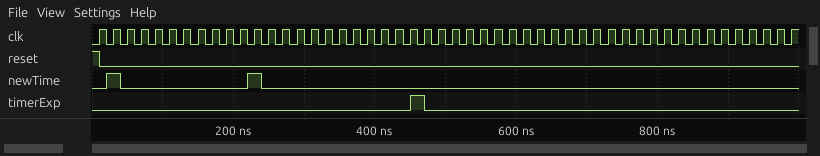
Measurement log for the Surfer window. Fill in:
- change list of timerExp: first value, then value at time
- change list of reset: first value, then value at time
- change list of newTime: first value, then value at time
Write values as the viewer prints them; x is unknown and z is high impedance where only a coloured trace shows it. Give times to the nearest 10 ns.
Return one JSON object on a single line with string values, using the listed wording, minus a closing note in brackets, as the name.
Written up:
{"change list of timerExp: first value, then value at time": "0, 1 at 450 ns, 0 at 470 ns", "change list of reset: first value, then value at time": "1, 0 at 10 ns", "change list of newTime: first value, then value at time": "0, 1 at 20 ns, 0 at 40 ns, 1 at 220 ns, 0 at 240 ns"}
